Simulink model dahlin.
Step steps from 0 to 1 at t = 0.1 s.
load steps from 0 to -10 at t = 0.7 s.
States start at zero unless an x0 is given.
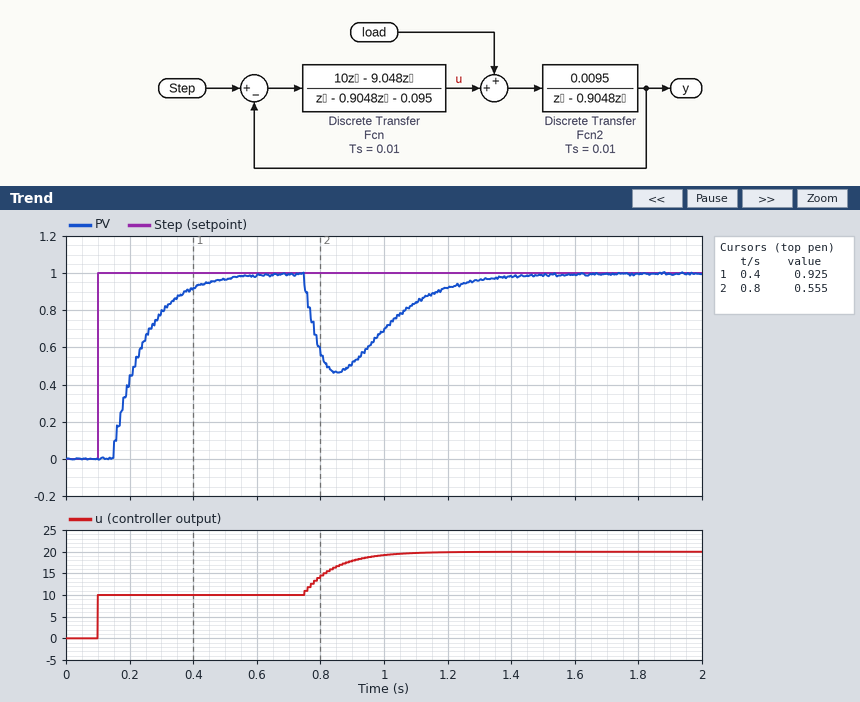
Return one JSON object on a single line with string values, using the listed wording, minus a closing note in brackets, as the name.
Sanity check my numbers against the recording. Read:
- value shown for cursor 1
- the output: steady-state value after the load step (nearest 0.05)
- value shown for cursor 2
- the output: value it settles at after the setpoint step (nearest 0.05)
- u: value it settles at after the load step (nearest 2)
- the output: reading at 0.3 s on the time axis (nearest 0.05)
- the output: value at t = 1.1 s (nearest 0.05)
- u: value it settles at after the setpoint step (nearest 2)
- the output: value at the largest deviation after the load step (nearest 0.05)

{"value shown for cursor 1": "0.925", "the output: steady-state value after the load step": "1.00", "value shown for cursor 2": "0.555", "the output: value it settles at after the setpoint step": "1.00", "u: value it settles at after the load step": "20", "the output: reading at 0.3 s on the time axis": "0.80", "the output: value at t = 1.1 s": "0.85", "u: value it settles at after the setpoint step": "10", "the output: value at the largest deviation after the load step": "0.45"}
